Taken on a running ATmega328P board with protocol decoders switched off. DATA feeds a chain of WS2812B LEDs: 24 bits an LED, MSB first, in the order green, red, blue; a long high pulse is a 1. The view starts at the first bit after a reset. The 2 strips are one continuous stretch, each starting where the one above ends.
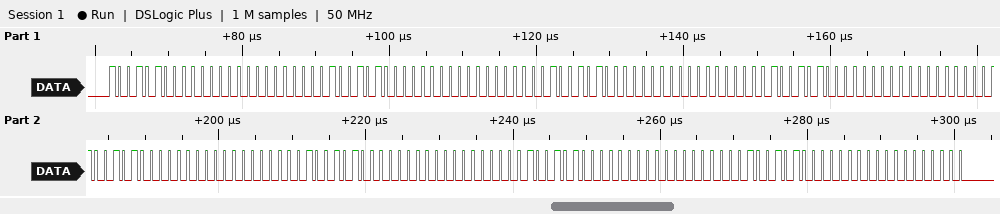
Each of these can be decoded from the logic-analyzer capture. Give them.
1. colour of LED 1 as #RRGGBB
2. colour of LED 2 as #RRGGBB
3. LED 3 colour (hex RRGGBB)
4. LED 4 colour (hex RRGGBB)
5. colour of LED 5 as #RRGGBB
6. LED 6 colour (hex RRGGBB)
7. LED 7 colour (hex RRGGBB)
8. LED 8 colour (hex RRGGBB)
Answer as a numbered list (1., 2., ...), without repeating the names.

1. #009400
2. #009400
3. #009400
4. #009400
5. #009400
6. #009400
7. #009400
8. #009400
